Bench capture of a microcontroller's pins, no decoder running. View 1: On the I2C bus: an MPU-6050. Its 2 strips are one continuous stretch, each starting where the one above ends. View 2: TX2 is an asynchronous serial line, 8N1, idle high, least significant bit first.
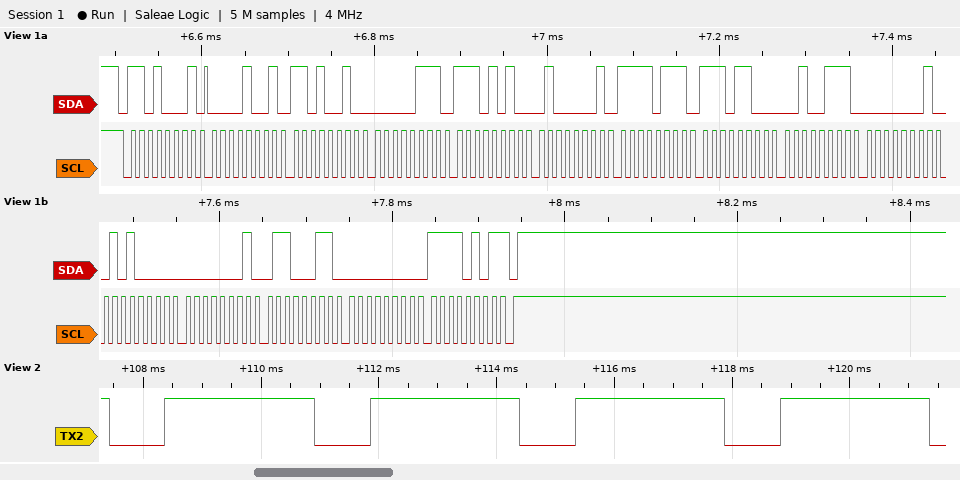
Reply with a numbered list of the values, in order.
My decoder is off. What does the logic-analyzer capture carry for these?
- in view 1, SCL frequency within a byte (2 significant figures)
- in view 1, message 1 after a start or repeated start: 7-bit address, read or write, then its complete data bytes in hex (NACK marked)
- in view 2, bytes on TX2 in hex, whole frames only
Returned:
1. 100 kHz
2. 0x68 read: 09 D2 07 EA 41 F7 EC 27 01 50 01 63 00 F5 NACK
3. 00 00 00 00
